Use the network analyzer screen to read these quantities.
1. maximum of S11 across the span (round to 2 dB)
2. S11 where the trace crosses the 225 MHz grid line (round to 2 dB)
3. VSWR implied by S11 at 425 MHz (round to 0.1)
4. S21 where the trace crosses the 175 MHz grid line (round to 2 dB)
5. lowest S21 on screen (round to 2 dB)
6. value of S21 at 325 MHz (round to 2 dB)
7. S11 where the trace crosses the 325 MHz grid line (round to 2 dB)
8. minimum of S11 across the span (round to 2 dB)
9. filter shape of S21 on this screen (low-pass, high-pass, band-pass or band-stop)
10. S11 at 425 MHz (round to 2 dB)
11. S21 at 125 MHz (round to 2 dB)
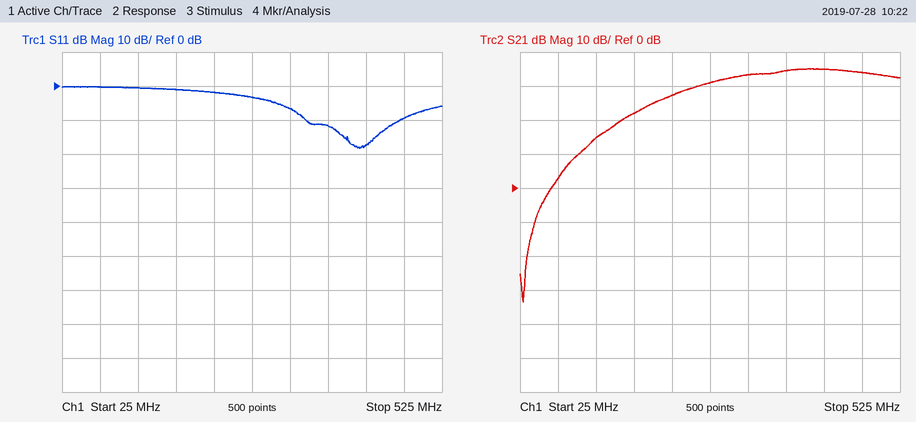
0 dB
-2 dB
1.3
22 dB
-34 dB
34 dB
-6 dB
-18 dB
high-pass
-18 dB
14 dB
